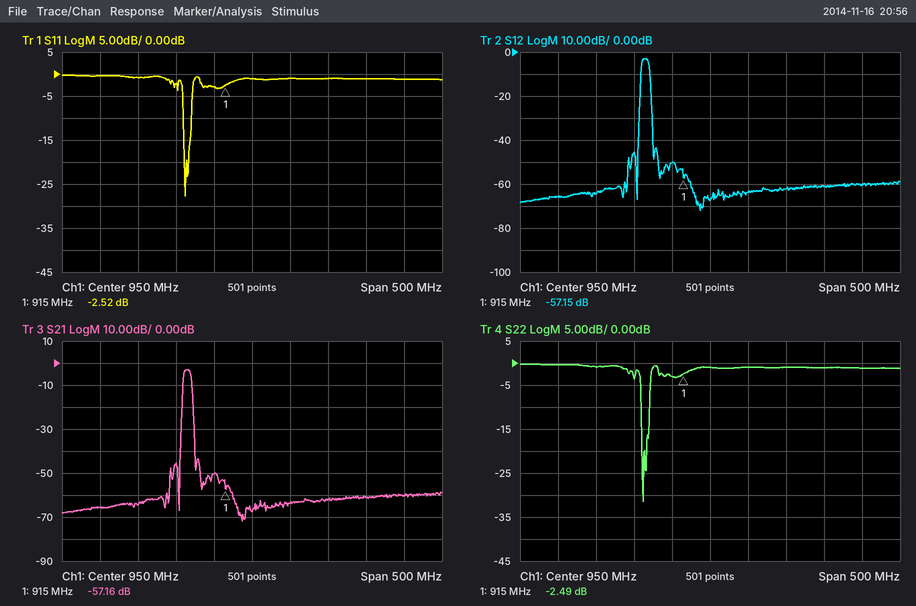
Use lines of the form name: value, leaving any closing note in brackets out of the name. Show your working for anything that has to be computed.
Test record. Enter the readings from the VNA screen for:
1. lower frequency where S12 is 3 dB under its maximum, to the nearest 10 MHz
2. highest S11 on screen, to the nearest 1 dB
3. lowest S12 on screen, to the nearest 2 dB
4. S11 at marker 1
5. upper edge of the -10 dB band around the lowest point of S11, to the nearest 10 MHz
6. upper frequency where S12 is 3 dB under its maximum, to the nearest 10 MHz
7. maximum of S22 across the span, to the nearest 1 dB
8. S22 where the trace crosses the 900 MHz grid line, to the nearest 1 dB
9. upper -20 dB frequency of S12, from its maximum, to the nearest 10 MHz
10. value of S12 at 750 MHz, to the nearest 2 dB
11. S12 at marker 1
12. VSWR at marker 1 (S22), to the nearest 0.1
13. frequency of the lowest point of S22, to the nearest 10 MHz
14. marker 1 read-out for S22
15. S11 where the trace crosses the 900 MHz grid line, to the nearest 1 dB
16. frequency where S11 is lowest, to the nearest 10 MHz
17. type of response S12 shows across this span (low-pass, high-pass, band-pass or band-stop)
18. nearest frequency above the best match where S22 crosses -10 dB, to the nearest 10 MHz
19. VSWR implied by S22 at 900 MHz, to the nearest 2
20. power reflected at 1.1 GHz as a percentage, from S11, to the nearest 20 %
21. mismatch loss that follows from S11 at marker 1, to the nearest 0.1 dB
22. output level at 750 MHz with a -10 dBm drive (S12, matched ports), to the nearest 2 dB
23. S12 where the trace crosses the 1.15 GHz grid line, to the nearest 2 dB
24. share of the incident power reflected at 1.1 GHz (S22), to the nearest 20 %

lower frequency where S12 is 3 dB under its maximum, to the nearest 10 MHz: 860 MHz
highest S11 on screen, to the nearest 1 dB: 0 dB
lowest S12 on screen, to the nearest 2 dB: -72 dB
S11 at marker 1: -2.52 dB
upper edge of the -10 dB band around the lowest point of S11, to the nearest 10 MHz: 870 MHz
upper frequency where S12 is 3 dB under its maximum, to the nearest 10 MHz: 870 MHz
maximum of S22 across the span, to the nearest 1 dB: 0 dB
S22 where the trace crosses the 900 MHz grid line, to the nearest 1 dB: -3 dB
upper -20 dB frequency of S12, from its maximum, to the nearest 10 MHz: 870 MHz
value of S12 at 750 MHz, to the nearest 2 dB: -66 dB
S12 at marker 1: -57.15 dB
VSWR at marker 1 (S22), to the nearest 0.1: (1 + 0.7508)/(1 − 0.7508) ≈ 7.0
frequency of the lowest point of S22, to the nearest 10 MHz: 860 MHz
marker 1 read-out for S22: -2.49 dB
S11 where the trace crosses the 900 MHz grid line, to the nearest 1 dB: -3 dB
frequency where S11 is lowest, to the nearest 10 MHz: 860 MHz
type of response S12 shows across this span: band-pass
nearest frequency above the best match where S22 crosses -10 dB, to the nearest 10 MHz: 870 MHz
VSWR implied by S22 at 900 MHz, to the nearest 2: |Γ| = 10^(-3/20) = 0.7079; VSWR = (1 + 0.7079)/(1 − 0.7079) ≈ 6
power reflected at 1.1 GHz as a percentage, from S11, to the nearest 20 %: 10^(-1/10) ≈ 79.4 %, so 80 % to the nearest 20 %
mismatch loss that follows from S11 at marker 1, to the nearest 0.1 dB: −10 log10(1 − 10^(-2.52/10)) ≈ 3.6 dB
output level at 750 MHz with a -10 dBm drive (S12, matched ports), to the nearest 2 dB: -10 dBm + (-66 dB) = -76 dBm
S12 where the trace crosses the 1.15 GHz grid line, to the nearest 2 dB: -60 dB
share of the incident power reflected at 1.1 GHz (S22), to the nearest 20 %: 10^(-1/10) ≈ 79.4 %, so 80 % to the nearest 20 %
